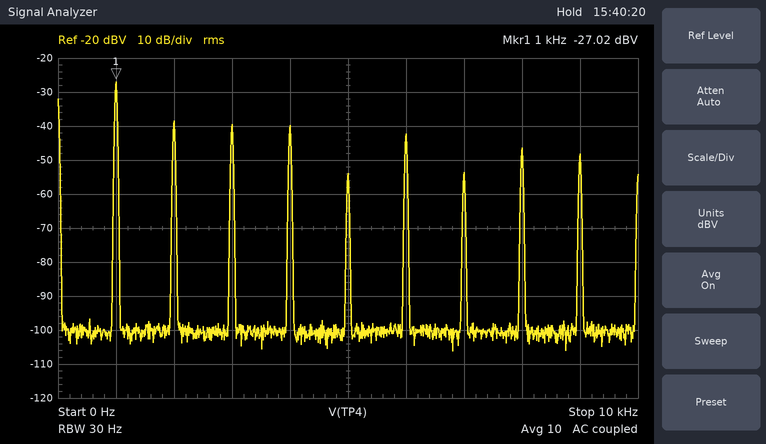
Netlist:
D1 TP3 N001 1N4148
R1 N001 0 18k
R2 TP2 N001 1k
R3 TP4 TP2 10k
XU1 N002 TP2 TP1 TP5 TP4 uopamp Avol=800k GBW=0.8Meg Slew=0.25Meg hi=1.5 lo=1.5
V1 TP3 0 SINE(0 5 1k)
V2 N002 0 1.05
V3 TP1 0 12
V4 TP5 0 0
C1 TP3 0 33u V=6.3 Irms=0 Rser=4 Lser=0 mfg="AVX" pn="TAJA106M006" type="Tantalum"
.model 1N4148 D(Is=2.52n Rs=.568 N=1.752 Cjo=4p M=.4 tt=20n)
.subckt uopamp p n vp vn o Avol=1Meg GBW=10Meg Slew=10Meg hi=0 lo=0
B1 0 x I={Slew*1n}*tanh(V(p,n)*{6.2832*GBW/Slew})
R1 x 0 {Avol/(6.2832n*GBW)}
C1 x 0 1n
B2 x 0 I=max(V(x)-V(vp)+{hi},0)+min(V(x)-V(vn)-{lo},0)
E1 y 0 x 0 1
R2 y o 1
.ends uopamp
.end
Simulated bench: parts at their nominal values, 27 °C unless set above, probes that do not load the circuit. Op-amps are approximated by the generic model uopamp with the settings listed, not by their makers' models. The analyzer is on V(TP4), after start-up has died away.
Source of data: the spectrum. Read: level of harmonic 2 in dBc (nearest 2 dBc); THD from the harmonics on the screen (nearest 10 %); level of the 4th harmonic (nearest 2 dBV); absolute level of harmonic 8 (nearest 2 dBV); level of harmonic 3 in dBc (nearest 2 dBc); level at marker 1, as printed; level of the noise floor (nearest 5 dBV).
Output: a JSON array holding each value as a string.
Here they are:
["-12 dBc", "50 %", "-40 dBV", "-46 dBV", "-12 dBc", "-27.02 dBV", "-100 dBV"]
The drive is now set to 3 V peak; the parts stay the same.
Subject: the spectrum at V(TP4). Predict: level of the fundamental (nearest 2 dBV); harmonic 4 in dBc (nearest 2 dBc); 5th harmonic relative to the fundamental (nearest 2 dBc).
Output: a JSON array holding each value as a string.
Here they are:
["-28 dBV", "-12 dBc", "-16 dBc"]
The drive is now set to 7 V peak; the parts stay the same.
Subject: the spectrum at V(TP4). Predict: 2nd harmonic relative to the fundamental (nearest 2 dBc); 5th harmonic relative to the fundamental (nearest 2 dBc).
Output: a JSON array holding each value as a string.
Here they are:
["-14 dBc", "-18 dBc"]
